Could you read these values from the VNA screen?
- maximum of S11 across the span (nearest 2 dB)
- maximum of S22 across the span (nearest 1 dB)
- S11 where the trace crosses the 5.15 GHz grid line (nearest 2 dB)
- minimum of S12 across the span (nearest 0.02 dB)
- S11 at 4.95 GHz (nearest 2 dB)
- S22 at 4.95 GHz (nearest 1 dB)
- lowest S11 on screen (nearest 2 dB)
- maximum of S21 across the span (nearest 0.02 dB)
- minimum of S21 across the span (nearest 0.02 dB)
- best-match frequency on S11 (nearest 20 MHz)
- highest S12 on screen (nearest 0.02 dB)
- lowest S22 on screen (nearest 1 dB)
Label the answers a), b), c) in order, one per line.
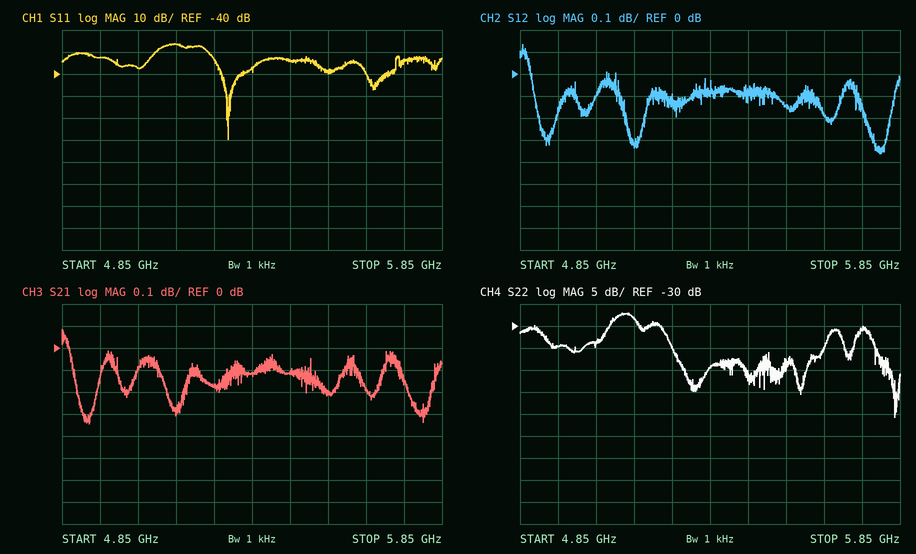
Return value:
a) -26 dB
b) -27 dB
c) -26 dB
d) -0.36 dB
e) -32 dB
f) -35 dB
g) -70 dB
h) 0.08 dB
i) -0.34 dB
j) 5.28 GHz
k) 0.14 dB
l) -51 dB
